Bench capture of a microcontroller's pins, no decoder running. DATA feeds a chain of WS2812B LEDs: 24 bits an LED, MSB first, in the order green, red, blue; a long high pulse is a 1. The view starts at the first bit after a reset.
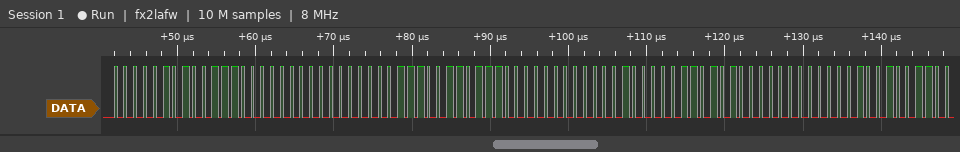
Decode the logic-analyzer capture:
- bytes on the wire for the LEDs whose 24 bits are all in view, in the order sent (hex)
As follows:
05 38 00 07 37 00 08 35 00
